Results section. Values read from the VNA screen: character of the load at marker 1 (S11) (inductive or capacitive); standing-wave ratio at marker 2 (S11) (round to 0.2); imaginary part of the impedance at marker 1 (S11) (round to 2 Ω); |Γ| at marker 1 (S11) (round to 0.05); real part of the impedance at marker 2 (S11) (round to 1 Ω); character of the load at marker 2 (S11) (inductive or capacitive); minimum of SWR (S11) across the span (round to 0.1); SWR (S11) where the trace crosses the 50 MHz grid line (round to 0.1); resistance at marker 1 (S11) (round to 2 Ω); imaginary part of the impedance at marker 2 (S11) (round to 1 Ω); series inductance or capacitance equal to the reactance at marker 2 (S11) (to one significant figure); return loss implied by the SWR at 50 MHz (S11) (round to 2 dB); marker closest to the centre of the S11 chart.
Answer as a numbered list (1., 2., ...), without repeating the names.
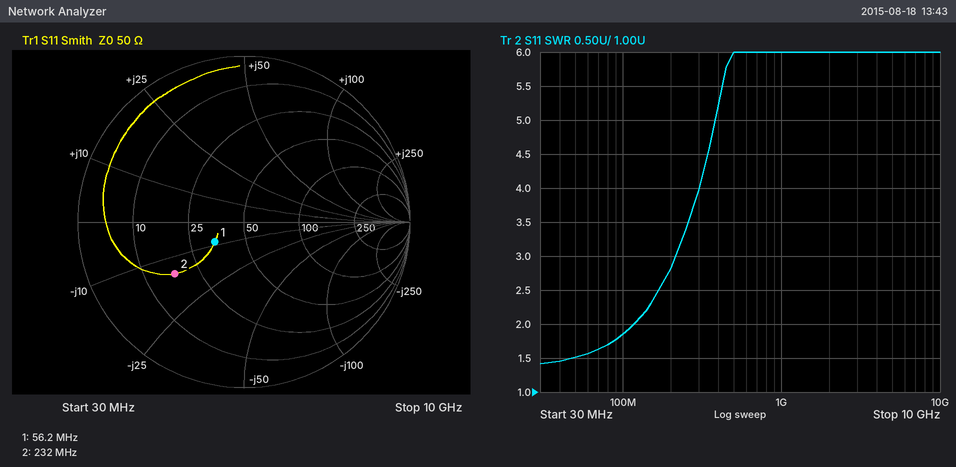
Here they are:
1. capacitive
2. 3.2
3. -8 Ω
4. 0.20
5. 17 Ω
6. capacitive
7. 1.4
8. 1.5
9. 34 Ω
10. -15 Ω
11. 50 pF
12. 14 dB
13. marker 1
